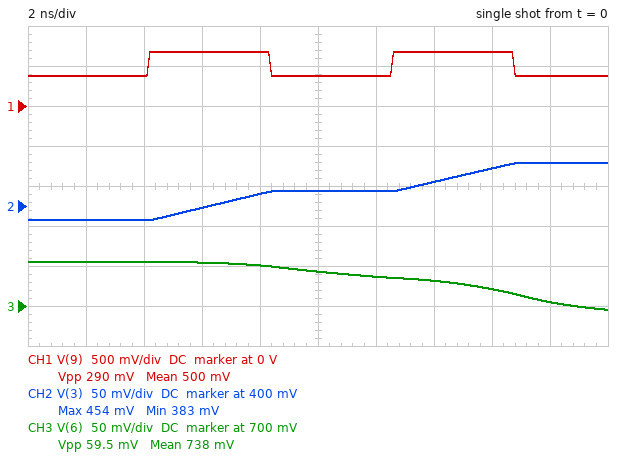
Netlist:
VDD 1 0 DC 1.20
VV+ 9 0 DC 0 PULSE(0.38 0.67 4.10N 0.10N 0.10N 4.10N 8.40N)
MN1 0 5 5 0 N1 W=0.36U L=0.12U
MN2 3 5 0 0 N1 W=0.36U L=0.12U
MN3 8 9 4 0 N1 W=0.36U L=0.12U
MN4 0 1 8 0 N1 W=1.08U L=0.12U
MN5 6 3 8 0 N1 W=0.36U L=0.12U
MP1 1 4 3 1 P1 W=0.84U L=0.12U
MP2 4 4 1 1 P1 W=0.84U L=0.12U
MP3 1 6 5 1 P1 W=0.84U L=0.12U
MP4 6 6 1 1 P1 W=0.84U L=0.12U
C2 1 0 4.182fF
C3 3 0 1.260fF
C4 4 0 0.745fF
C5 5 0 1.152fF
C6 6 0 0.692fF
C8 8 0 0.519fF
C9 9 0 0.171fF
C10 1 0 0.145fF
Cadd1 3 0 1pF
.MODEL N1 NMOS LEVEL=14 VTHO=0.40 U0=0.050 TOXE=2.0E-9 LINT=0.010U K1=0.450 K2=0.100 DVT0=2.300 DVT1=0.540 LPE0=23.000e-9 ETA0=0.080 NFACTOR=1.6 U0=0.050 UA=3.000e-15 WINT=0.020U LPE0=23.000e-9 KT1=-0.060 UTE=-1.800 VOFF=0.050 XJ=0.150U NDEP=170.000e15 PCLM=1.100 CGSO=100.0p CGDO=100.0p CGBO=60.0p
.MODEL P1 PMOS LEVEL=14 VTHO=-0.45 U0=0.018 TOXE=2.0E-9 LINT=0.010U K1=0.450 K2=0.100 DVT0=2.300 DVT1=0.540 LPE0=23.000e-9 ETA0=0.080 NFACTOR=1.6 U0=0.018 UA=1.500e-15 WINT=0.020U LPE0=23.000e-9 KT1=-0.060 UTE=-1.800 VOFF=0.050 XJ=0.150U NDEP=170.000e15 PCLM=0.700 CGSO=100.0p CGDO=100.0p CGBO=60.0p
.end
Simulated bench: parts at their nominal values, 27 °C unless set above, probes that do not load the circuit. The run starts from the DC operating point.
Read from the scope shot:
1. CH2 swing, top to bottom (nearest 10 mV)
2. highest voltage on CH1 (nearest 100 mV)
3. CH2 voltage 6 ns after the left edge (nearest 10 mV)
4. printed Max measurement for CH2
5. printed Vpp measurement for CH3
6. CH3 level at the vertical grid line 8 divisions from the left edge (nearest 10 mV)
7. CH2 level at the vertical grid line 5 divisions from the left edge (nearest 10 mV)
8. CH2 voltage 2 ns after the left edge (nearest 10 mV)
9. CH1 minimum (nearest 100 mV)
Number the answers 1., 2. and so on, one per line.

1. 70 mV
2. 700 mV
3. 400 mV
4. 454 mV
5. 59.5 mV
6. 720 mV
7. 420 mV
8. 380 mV
9. 400 mV
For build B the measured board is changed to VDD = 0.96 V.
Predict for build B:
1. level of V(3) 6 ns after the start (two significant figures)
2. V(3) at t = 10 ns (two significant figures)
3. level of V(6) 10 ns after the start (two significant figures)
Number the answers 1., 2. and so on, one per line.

1. 390 mV
2. 400 mV
3. 520 mV
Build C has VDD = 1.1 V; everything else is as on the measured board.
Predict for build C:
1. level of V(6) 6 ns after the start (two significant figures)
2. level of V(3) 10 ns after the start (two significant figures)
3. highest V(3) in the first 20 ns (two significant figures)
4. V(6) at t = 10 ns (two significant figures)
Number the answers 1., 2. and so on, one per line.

1. 660 mV
2. 410 mV
3. 440 mV
4. 650 mV
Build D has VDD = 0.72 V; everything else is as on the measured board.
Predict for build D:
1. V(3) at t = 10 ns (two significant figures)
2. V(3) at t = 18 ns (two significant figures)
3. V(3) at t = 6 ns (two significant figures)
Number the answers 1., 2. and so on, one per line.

1. 390 mV
2. 400 mV
3. 380 mV
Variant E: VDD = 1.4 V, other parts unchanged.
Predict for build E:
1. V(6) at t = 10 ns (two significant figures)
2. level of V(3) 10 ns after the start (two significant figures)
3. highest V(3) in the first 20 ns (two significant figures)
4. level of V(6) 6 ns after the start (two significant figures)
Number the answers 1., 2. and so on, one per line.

1. 920 mV
2. 430 mV
3. 480 mV
4. 950 mV
